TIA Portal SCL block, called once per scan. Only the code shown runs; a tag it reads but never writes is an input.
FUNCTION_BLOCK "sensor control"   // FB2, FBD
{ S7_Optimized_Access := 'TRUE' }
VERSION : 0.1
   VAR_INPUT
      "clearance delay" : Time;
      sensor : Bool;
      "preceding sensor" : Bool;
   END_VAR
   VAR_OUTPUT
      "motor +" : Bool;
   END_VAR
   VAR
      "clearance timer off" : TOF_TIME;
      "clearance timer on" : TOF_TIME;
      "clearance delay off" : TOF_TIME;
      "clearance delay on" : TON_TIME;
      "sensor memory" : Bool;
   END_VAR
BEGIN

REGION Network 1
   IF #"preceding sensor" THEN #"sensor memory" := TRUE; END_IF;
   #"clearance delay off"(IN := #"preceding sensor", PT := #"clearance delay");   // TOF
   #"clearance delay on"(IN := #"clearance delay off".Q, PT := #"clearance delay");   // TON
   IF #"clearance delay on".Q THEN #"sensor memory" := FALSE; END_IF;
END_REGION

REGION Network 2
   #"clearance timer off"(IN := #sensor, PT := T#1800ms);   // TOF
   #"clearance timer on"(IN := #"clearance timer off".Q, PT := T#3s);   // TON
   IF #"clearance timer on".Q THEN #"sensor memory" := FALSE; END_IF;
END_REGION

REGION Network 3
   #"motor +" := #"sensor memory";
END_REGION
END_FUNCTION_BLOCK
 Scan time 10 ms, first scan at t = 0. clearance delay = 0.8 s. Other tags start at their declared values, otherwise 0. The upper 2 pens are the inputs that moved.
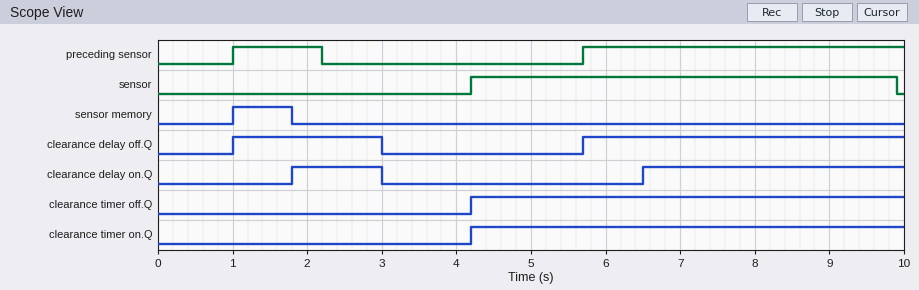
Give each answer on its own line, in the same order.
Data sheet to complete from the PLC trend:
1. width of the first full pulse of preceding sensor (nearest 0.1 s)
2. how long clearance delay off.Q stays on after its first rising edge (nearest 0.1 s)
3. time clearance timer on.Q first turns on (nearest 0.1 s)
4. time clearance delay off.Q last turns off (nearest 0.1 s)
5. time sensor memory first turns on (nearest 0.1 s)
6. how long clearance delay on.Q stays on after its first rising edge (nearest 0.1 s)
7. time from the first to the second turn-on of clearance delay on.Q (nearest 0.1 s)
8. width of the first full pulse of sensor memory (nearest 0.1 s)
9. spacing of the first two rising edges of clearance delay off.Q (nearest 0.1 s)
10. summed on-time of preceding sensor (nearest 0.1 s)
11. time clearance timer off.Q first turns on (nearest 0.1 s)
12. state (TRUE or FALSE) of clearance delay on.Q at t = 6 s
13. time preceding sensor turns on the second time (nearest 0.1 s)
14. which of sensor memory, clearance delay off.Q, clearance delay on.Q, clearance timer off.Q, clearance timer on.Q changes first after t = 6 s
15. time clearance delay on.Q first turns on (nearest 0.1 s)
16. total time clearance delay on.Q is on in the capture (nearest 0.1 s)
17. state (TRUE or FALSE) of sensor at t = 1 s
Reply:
1.2 s
2.0 s
4.2 s
3.0 s
1.0 s
1.2 s
4.7 s
0.8 s
4.7 s
5.5 s
4.2 s
FALSE
5.7 s
clearance delay on.Q
1.8 s
4.7 s
FALSE
